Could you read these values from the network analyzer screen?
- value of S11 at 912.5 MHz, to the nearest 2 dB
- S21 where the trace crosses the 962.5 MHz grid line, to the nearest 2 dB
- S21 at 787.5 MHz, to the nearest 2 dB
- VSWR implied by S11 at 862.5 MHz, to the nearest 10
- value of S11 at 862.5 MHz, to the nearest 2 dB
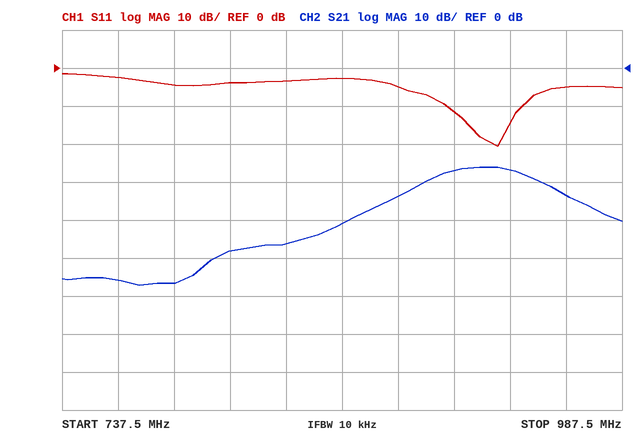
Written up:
-12 dB
-34 dB
-56 dB
10
-2 dB
